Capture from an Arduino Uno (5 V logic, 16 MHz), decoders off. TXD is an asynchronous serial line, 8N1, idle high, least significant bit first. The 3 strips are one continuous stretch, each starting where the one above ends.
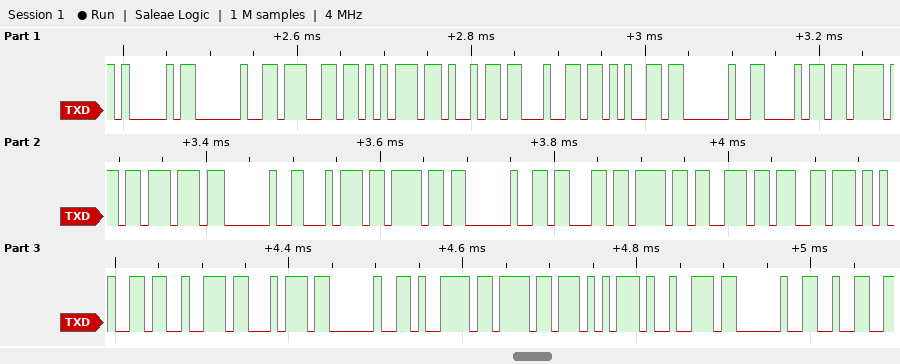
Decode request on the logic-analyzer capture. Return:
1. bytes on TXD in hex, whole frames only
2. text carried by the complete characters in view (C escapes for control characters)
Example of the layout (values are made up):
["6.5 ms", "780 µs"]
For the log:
["41 20 67 75 69 64 65 20 68 6F 77 20 74 6F 20 63 6F 6E 76 65 72 74 20 79 6F 75 72 20 32", "\"A guide how to convert your 2\""]
